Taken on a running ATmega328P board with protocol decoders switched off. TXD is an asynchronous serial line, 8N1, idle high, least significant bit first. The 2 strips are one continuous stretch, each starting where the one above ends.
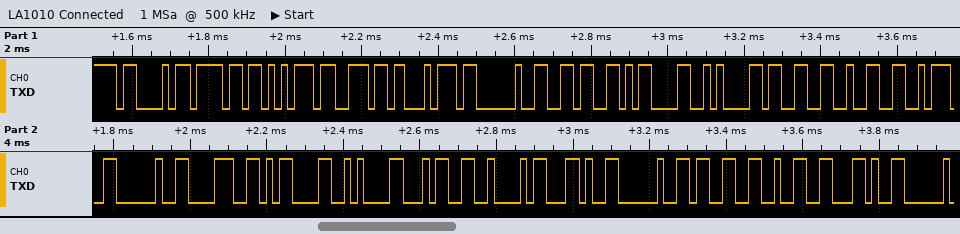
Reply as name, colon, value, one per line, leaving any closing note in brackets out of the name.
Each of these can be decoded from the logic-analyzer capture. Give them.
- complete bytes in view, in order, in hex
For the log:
complete bytes in view, in order, in hex: 43 6F 75 6E 74 20 36 0D 0A 33 32 3A 20 38 0D 0A 34 42 2C 20 33 32 2C
